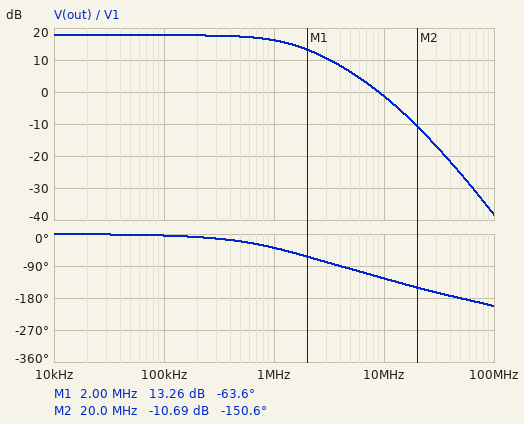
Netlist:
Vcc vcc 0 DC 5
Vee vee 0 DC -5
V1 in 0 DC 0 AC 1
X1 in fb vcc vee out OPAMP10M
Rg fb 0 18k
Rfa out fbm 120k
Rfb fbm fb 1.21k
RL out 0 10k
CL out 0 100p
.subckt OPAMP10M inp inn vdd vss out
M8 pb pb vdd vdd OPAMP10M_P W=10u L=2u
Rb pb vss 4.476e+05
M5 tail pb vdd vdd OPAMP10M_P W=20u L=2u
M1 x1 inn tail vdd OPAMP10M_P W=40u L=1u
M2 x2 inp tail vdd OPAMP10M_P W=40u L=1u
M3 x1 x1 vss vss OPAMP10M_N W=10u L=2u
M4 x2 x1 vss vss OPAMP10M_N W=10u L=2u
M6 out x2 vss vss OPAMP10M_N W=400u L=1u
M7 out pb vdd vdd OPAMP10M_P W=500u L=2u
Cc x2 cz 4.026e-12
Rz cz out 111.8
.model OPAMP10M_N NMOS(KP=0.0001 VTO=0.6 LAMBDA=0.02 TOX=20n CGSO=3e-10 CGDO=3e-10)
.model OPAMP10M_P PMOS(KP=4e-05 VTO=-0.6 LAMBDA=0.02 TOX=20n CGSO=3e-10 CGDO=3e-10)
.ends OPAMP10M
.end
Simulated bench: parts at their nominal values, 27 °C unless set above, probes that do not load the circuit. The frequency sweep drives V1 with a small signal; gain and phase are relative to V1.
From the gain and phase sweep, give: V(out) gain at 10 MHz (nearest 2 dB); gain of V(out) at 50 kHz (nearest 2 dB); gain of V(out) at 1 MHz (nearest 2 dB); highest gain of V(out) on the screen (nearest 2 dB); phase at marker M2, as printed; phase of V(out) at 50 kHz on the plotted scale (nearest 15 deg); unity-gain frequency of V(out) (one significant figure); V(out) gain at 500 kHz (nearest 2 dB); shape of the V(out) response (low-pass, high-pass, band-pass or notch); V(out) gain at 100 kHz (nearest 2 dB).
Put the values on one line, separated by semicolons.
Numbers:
-2 dB; 18 dB; 16 dB; 18 dB; -150.6 deg; 0 deg; 9 MHz; 18 dB; low-pass; 18 dB
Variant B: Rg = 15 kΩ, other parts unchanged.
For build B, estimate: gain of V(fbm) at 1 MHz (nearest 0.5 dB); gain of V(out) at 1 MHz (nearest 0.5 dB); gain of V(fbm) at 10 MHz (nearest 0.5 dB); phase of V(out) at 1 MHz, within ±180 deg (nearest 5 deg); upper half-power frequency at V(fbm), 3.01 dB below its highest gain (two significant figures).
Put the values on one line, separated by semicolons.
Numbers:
-1.5 dB; 17.0 dB; -22.0 dB; -45 deg; 1.2 MHz
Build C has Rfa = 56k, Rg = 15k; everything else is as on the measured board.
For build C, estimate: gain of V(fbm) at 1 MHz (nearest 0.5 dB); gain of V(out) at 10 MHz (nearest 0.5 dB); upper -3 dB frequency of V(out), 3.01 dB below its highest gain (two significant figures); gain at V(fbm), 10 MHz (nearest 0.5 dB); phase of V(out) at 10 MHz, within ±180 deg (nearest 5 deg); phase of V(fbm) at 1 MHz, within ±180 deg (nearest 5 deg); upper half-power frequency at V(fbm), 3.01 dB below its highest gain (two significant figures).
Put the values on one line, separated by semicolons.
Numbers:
0 dB; -1.0 dB; 2.6 MHz; -15.0 dB; -120 deg; -25 deg; 2.5 MHz
